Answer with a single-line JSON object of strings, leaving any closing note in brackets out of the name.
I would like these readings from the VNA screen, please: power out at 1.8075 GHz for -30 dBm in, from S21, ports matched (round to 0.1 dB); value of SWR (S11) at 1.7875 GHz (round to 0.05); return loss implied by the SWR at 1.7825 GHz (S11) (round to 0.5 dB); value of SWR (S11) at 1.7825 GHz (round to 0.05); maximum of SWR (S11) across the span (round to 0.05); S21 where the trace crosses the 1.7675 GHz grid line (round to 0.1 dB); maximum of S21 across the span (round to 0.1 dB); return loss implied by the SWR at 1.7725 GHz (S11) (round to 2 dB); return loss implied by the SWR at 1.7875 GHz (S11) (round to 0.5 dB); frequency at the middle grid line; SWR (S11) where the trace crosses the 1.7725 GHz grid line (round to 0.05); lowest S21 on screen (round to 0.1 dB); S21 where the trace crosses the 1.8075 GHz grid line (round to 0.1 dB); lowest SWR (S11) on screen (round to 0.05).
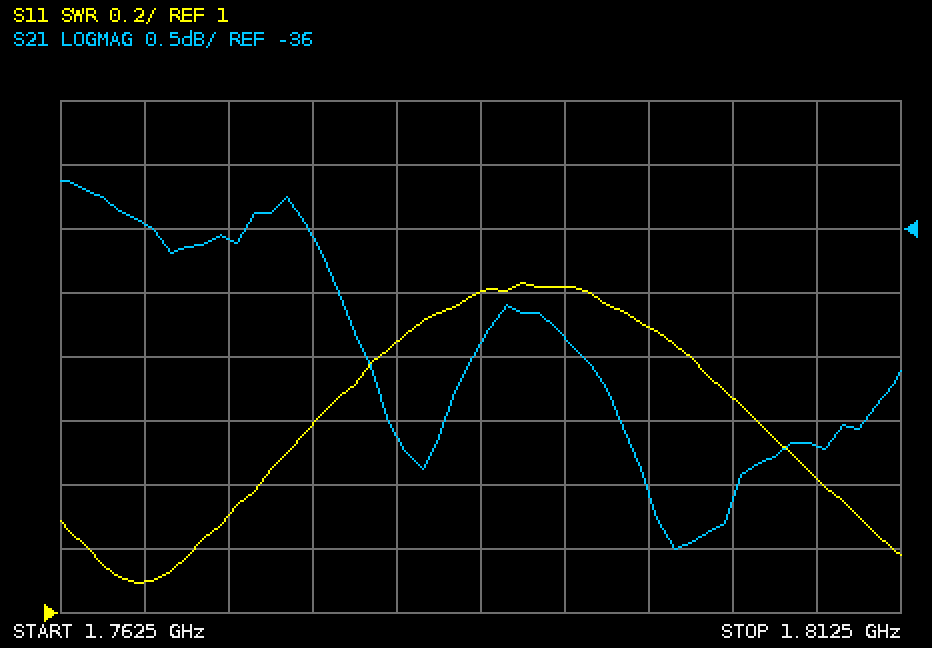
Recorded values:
{"power out at 1.8075 GHz for -30 dBm in, from S21, ports matched": "-67.7 dBm", "value of SWR (S11) at 1.7875 GHz": "2.00", "return loss implied by the SWR at 1.7825 GHz (S11)": "10.5 dB", "value of SWR (S11) at 1.7825 GHz": "1.85", "maximum of SWR (S11) across the span": "2.05", "S21 where the trace crosses the 1.7675 GHz grid line": "-36.0 dB", "maximum of S21 across the span": "-35.6 dB", "return loss implied by the SWR at 1.7725 GHz (S11)": "18 dB", "return loss implied by the SWR at 1.7875 GHz (S11)": "9.5 dB", "frequency at the middle grid line": "1.7875 GHz", "SWR (S11) where the trace crosses the 1.7725 GHz grid line": "1.30", "lowest S21 on screen": "-38.5 dB", "S21 where the trace crosses the 1.8075 GHz grid line": "-37.7 dB", "lowest SWR (S11) on screen": "1.10"}
